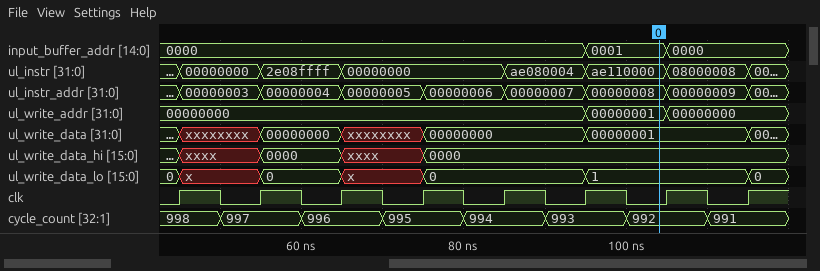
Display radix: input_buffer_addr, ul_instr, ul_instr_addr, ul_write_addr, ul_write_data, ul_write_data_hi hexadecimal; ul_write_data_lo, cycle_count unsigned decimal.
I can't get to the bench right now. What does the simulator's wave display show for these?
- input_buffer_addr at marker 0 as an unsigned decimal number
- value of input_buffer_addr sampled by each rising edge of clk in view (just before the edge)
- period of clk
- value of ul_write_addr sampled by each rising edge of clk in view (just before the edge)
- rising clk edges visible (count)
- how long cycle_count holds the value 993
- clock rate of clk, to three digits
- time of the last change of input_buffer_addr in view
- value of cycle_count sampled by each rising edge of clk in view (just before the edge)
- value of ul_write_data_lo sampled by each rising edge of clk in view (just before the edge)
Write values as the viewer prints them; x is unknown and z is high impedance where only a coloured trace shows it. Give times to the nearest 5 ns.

1
0000, 0000, 0000, 0000, 0000, 0000, 0001, 0000
10 ns
00000000, 00000000, 00000000, 00000000, 00000000, 00000000, 00000001, 00000000
8
10 ns
100 MHz
105 ns
998, 997, 996, 995, 994, 993, 992, 991
0, x, 0, x, 0, 0, 1, 1
